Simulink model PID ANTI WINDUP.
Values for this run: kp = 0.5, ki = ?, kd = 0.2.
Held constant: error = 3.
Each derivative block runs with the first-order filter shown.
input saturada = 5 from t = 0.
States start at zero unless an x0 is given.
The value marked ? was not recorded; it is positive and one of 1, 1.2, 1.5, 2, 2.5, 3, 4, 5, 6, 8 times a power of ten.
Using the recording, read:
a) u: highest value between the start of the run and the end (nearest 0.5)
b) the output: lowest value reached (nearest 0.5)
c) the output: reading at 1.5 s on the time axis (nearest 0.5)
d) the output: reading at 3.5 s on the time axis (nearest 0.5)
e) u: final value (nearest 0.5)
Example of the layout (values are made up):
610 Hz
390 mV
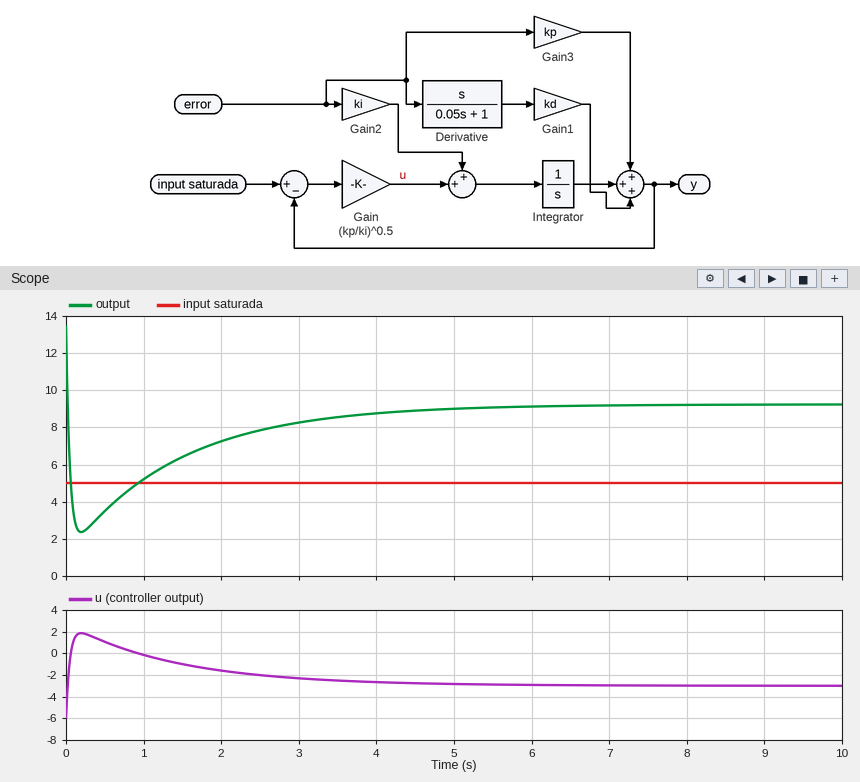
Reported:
2.0
2.5
6.5
8.5
-3.0
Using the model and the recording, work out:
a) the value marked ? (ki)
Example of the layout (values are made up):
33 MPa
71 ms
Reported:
1
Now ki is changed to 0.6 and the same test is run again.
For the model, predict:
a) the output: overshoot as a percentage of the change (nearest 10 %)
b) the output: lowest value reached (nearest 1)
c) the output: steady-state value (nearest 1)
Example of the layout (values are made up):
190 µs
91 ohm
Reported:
70 %
2
7
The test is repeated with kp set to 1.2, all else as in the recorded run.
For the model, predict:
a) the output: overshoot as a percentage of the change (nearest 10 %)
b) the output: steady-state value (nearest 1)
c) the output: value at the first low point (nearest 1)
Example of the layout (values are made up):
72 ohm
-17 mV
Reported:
50 %
8
4
